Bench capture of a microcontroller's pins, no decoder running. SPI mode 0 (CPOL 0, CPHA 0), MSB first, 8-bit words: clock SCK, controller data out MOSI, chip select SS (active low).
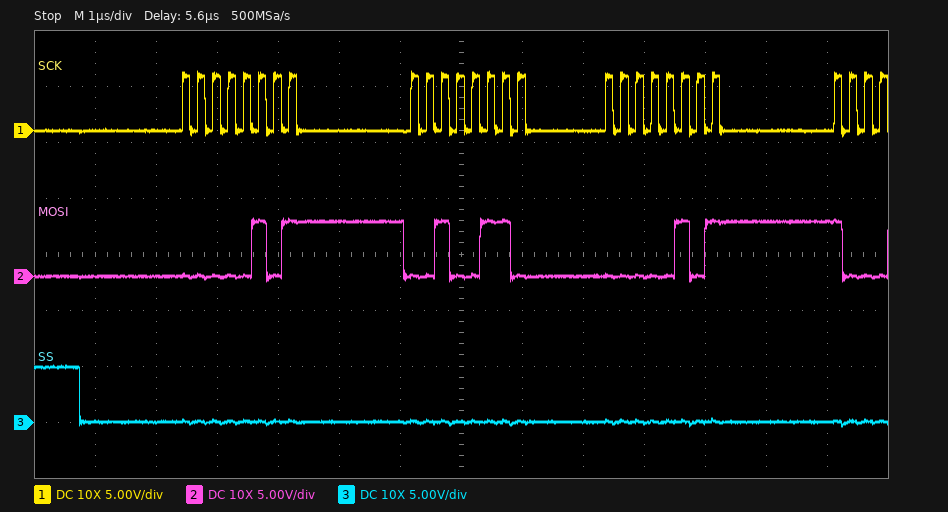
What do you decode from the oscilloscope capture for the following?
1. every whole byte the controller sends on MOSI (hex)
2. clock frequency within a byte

05 26 05
4 MHz
